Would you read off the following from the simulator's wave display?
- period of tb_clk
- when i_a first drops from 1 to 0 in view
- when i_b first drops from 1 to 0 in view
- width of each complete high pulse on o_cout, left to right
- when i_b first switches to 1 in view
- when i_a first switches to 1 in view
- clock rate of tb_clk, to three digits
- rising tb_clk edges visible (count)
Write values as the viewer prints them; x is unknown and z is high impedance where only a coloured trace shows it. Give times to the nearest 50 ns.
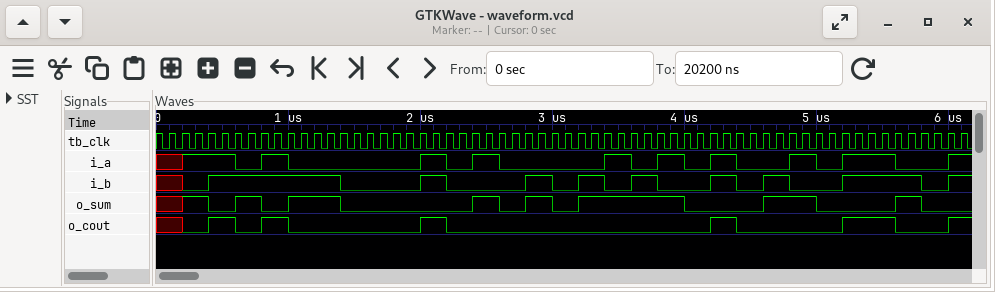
100 ns
600 ns
1400 ns
200 ns, 200 ns, 200 ns, 200 ns, 400 ns
400 ns
200 ns
10.0 MHz
61
